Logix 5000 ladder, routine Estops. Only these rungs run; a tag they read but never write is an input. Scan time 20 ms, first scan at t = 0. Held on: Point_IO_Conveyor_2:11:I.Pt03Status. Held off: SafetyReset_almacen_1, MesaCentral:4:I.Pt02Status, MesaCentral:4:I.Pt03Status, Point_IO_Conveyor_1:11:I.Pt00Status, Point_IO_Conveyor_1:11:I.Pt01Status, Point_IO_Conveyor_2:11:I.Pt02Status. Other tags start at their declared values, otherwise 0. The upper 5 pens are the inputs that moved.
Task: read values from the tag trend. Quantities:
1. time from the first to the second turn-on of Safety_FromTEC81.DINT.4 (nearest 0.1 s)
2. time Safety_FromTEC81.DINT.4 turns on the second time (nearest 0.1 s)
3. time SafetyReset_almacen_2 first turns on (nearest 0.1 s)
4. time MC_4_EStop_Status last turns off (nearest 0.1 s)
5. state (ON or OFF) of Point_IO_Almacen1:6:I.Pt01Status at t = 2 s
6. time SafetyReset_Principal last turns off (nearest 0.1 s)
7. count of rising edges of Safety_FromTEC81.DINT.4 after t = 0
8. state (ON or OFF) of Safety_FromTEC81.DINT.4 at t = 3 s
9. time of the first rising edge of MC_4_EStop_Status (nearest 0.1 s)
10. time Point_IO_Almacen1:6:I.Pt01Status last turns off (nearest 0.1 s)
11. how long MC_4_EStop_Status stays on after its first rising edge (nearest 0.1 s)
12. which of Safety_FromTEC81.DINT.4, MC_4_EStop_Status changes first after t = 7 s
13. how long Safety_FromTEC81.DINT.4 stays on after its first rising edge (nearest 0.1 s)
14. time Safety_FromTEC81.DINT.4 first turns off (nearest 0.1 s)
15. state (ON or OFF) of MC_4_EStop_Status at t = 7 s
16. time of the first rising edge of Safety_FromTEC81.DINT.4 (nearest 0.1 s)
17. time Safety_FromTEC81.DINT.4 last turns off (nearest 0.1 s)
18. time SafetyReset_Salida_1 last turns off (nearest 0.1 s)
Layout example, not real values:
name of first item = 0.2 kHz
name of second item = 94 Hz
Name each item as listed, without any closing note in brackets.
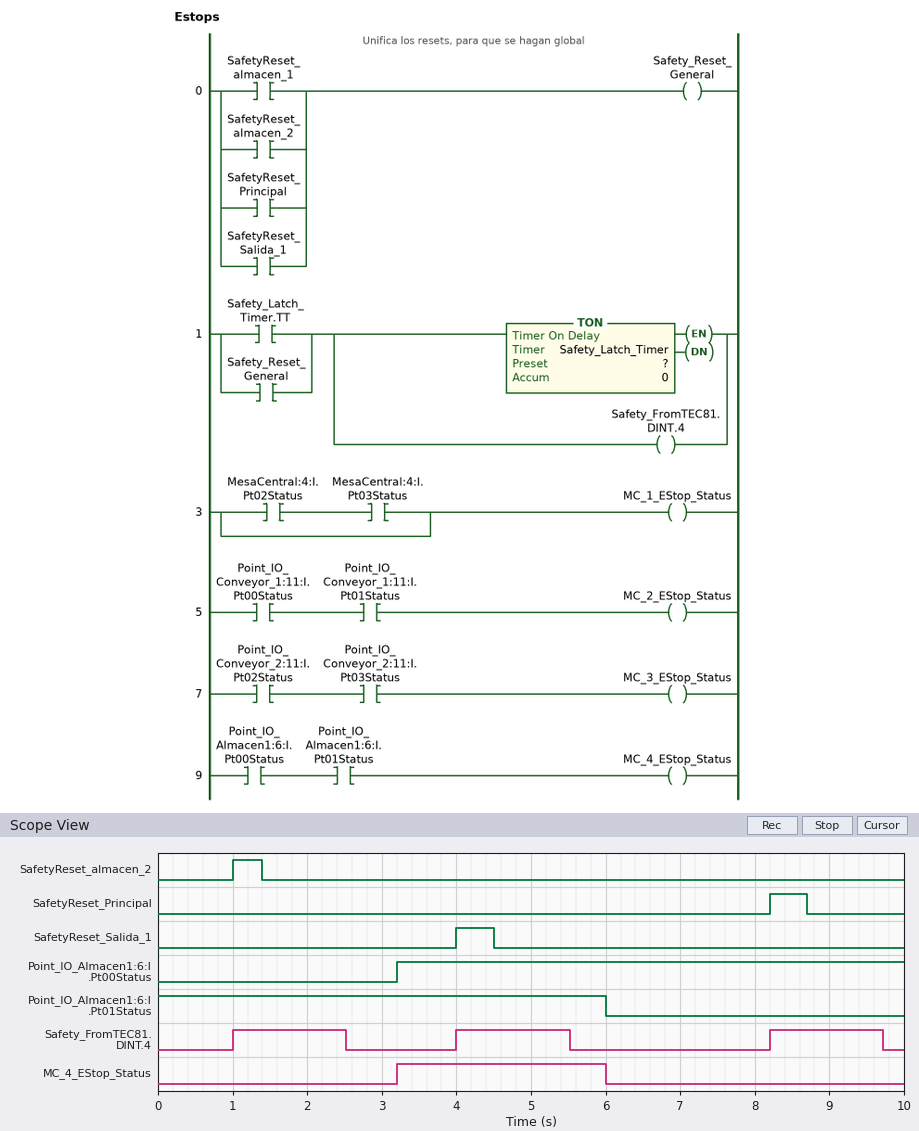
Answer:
time from the first to the second turn-on of Safety_FromTEC81.DINT.4 = 3.0 s
time Safety_FromTEC81.DINT.4 turns on the second time = 4.0 s
time SafetyReset_almacen_2 first turns on = 1.0 s
time MC_4_EStop_Status last turns off = 6.0 s
state (ON or OFF) of Point_IO_Almacen1:6:I.Pt01Status at t = 2 s = ON
time SafetyReset_Principal last turns off = 8.7 s
count of rising edges of Safety_FromTEC81.DINT.4 after t = 0 = 3
state (ON or OFF) of Safety_FromTEC81.DINT.4 at t = 3 s = OFF
time of the first rising edge of MC_4_EStop_Status = 3.2 s
time Point_IO_Almacen1:6:I.Pt01Status last turns off = 6.0 s
how long MC_4_EStop_Status stays on after its first rising edge = 2.8 s
which of Safety_FromTEC81.DINT.4, MC_4_EStop_Status changes first after t = 7 s = Safety_FromTEC81.DINT.4
how long Safety_FromTEC81.DINT.4 stays on after its first rising edge = 1.5 s
time Safety_FromTEC81.DINT.4 first turns off = 2.5 s
state (ON or OFF) of MC_4_EStop_Status at t = 7 s = OFF
time of the first rising edge of Safety_FromTEC81.DINT.4 = 1.0 s
time Safety_FromTEC81.DINT.4 last turns off = 9.7 s
time SafetyReset_Salida_1 last turns off = 4.5 s
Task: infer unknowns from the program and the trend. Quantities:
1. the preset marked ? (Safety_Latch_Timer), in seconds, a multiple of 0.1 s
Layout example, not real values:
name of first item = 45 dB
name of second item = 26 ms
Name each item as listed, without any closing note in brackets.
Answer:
the preset marked ? (Safety_Latch_Timer), in seconds, a multiple of 0.1 s = 1.5 s
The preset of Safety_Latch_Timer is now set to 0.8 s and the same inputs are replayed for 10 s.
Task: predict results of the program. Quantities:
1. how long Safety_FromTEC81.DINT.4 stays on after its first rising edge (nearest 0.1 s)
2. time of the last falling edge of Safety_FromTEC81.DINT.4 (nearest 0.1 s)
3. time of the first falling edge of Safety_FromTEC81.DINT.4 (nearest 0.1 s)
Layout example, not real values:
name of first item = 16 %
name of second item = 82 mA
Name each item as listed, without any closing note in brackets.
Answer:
how long Safety_FromTEC81.DINT.4 stays on after its first rising edge = 0.8 s
time of the last falling edge of Safety_FromTEC81.DINT.4 = 9.0 s
time of the first falling edge of Safety_FromTEC81.DINT.4 = 1.8 s
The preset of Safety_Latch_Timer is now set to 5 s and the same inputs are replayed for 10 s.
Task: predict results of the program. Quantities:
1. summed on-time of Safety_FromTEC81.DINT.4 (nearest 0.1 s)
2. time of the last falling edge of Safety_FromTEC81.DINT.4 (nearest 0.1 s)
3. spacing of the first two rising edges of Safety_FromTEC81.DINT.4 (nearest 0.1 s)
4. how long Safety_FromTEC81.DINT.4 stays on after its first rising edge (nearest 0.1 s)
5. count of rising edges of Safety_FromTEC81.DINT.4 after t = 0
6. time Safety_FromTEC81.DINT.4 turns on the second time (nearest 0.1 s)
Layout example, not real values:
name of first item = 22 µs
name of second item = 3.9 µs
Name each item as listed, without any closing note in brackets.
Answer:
summed on-time of Safety_FromTEC81.DINT.4 = 6.8 s
time of the last falling edge of Safety_FromTEC81.DINT.4 = 6.0 s
spacing of the first two rising edges of Safety_FromTEC81.DINT.4 = 7.2 s
how long Safety_FromTEC81.DINT.4 stays on after its first rising edge = 5.0 s
count of rising edges of Safety_FromTEC81.DINT.4 after t = 0 = 2
time Safety_FromTEC81.DINT.4 turns on the second time = 8.2 s
